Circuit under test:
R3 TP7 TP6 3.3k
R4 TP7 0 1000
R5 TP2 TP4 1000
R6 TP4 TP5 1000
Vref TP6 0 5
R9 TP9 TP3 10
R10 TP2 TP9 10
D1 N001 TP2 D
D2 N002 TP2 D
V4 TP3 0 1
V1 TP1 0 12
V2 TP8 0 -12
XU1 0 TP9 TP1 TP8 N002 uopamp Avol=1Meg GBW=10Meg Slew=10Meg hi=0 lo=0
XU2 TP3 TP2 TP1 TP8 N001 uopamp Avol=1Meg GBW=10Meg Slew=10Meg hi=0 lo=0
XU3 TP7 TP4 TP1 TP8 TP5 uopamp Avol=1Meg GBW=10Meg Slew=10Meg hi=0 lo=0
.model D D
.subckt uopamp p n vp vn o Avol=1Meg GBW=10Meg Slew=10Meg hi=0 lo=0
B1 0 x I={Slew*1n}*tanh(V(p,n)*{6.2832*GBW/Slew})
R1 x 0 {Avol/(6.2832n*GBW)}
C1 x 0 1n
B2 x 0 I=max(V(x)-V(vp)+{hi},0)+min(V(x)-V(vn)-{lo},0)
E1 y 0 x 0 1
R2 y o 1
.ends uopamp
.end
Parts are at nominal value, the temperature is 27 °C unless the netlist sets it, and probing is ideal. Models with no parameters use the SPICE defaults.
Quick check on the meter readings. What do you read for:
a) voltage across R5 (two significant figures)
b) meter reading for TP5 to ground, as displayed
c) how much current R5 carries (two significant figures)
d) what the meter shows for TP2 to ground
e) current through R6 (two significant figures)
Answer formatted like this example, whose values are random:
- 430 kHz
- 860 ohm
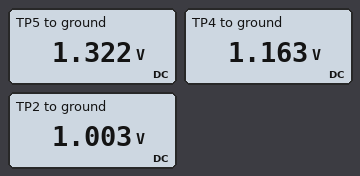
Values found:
- 160 mV
- 1.322 V
- 160 µA
- 1.003 V
- 160 µA
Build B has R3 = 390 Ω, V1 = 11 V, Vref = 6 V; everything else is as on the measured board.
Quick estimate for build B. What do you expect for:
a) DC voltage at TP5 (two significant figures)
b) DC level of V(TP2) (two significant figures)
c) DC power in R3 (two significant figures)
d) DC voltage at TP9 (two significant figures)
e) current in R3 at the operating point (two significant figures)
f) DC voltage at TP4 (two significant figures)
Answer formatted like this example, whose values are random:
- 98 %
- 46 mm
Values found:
- 7.6 V
- 1.1 V
- 7.3 mW
- 1.0 V
- 4.3 mA
- 4.3 V
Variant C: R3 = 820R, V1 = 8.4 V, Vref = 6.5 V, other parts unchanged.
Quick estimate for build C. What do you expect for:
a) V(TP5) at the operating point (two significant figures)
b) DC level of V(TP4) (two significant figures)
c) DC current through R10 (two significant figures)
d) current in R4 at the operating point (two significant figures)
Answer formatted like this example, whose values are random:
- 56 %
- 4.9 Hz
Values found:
- 6.1 V
- 3.6 V
- 2.5 mA
- 3.6 mA
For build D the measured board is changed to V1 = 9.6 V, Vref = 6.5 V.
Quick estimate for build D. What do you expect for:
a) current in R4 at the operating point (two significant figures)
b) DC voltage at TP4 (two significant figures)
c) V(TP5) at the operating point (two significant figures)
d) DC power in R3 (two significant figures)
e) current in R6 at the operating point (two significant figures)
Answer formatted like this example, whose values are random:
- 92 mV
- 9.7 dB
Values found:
- 1.5 mA
- 1.5 V
- 2.0 V
- 7.5 mW
- 500 µA
